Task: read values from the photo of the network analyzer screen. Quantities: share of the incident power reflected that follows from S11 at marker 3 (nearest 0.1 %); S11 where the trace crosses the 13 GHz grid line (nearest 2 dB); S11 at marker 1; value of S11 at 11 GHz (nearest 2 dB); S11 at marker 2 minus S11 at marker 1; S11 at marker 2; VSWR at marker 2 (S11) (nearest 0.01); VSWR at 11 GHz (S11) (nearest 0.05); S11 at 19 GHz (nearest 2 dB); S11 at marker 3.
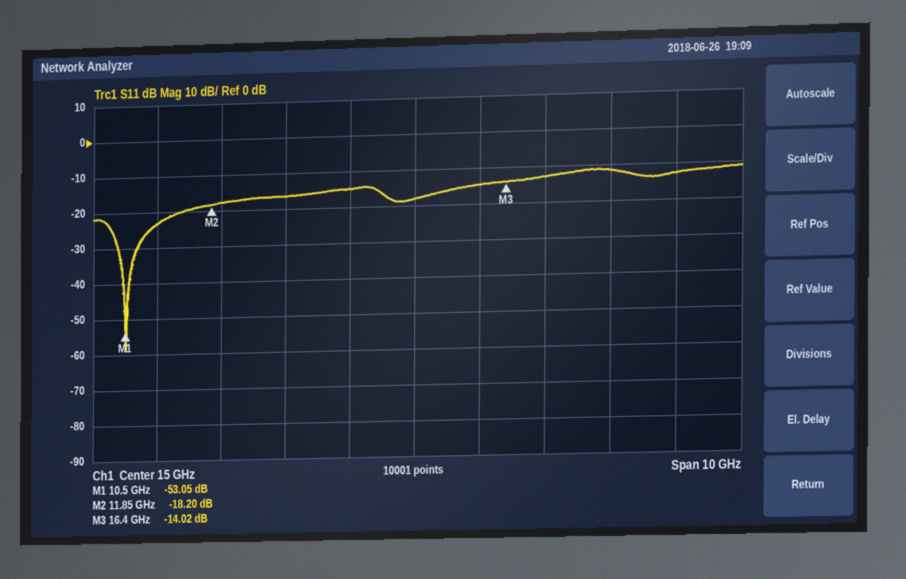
4.0 %
-16 dB
-53.05 dB
-24 dB
34.85 dB
-18.20 dB
1.28
1.15
-12 dB
-14.02 dB
